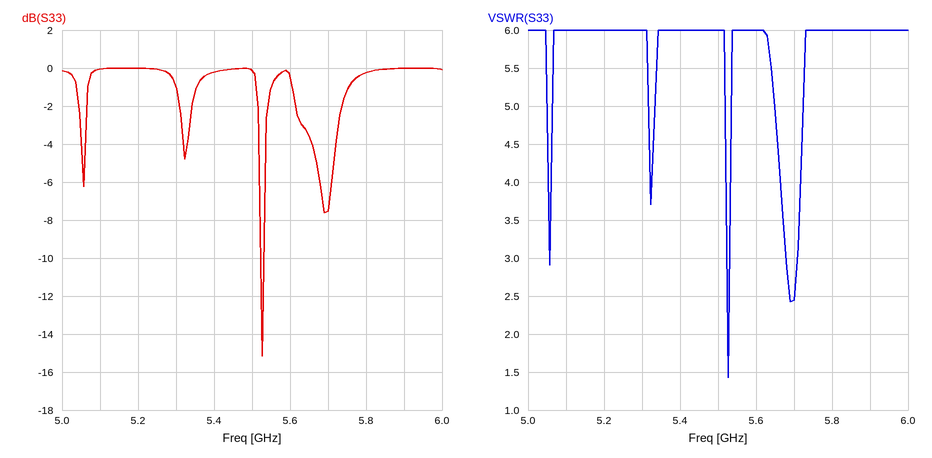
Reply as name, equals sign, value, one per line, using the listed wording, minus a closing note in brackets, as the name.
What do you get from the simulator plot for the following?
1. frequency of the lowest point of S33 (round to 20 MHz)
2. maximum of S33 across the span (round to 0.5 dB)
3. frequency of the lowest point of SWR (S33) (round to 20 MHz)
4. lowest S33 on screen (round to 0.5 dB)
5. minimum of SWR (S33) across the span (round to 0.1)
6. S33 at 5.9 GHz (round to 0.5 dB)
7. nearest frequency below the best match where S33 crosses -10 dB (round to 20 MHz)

frequency of the lowest point of S33 = 5.52 GHz
maximum of S33 across the span = 0.0 dB
frequency of the lowest point of SWR (S33) = 5.52 GHz
lowest S33 on screen = -15.0 dB
minimum of SWR (S33) across the span = 1.4
S33 at 5.9 GHz = 0.0 dB
nearest frequency below the best match where S33 crosses -10 dB = 5.52 GHz
